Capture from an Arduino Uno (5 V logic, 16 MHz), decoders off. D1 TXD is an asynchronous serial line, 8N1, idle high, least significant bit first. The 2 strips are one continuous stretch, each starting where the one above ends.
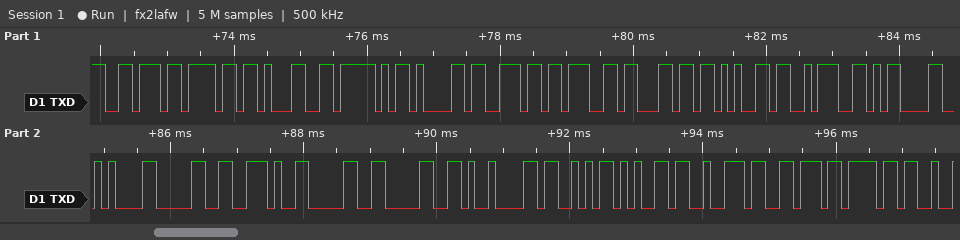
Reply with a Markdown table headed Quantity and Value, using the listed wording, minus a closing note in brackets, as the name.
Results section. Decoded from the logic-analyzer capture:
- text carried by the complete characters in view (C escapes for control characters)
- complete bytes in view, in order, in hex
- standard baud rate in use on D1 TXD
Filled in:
| Quantity | Value |
|---|---|
| text carried by the complete characters in view | "vo1_angle:\r\n0.00\tServo" |
| complete bytes in view, in order, in hex | 76 6F 31 5F 61 6E 67 6C 65 3A 0D 0A 30 2E 30 30 09 53 65 72 76 6F |
| standard baud rate in use on D1 TXD | 9600 baud |
